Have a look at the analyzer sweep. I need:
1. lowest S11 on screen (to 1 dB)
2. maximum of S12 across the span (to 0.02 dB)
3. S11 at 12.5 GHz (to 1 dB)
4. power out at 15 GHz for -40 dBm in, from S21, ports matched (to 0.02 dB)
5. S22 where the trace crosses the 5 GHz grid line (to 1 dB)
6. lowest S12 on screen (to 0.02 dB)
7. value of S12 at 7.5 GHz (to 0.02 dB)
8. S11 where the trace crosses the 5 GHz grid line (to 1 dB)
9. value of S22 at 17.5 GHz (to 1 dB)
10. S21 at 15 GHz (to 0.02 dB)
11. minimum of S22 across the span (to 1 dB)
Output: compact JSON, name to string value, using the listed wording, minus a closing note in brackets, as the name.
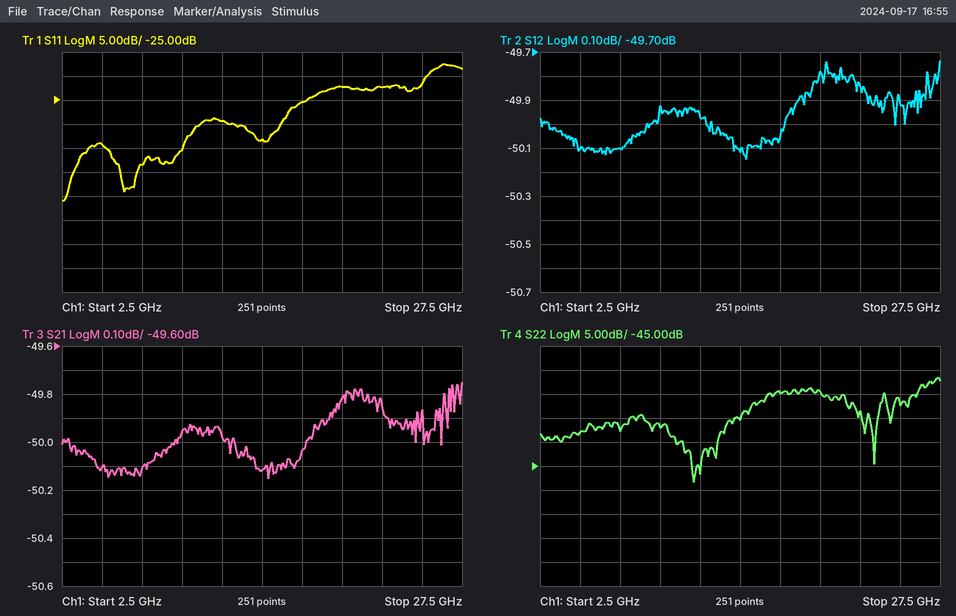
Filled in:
{"lowest S11 on screen": "-46 dB", "maximum of S12 across the span": "-49.74 dB", "S11 at 12.5 GHz": "-29 dB", "power out at 15 GHz for -40 dBm in, from S21, ports matched": "-90.12 dBm", "S22 where the trace crosses the 5 GHz grid line": "-38 dB", "lowest S12 on screen": "-50.14 dB", "value of S12 at 7.5 GHz": "-50.10 dB", "S11 where the trace crosses the 5 GHz grid line": "-34 dB", "value of S22 at 17.5 GHz": "-30 dB", "S21 at 15 GHz": "-50.12 dB", "minimum of S22 across the span": "-48 dB"}
